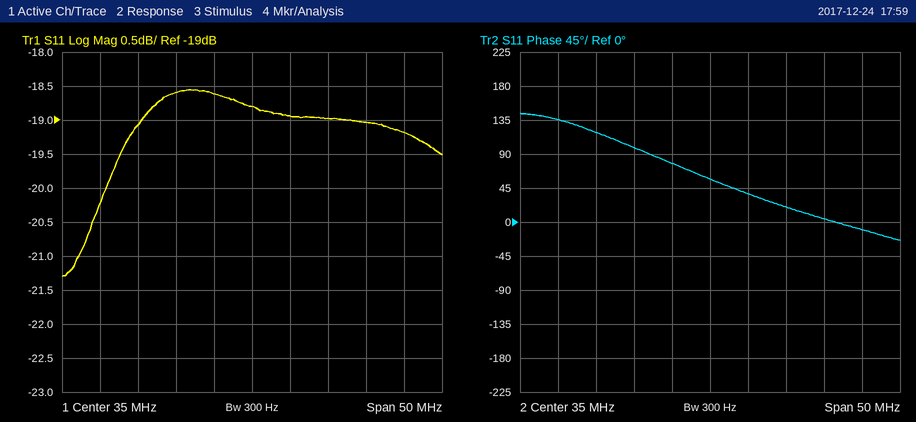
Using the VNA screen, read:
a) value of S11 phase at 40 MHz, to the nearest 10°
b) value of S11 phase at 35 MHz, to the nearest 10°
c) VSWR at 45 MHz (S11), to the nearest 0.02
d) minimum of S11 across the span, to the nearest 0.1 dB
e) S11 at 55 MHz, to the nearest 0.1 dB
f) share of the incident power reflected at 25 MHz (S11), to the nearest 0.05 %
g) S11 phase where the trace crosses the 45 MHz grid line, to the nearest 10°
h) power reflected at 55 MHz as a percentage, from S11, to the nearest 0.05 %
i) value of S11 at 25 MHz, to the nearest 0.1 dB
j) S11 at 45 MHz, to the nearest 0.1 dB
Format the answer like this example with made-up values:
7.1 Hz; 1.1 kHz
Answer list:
40°; 60°; 1.26; -21.3 dB; -19.2 dB; 1.40 %; 20°; 1.20 %; -18.6 dB; -19.0 dB
